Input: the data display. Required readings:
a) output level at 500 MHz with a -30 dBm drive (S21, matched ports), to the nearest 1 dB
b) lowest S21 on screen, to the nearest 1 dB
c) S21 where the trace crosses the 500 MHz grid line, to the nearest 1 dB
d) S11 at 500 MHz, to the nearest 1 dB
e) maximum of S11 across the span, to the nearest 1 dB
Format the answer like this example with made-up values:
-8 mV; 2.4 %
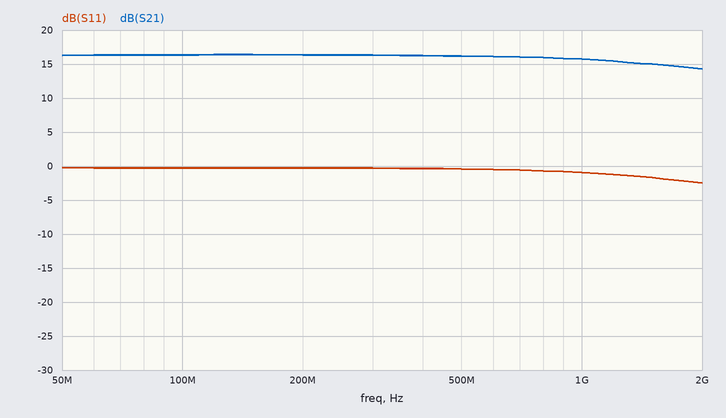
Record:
-14 dBm; 14 dB; 16 dB; 0 dB; 0 dB
